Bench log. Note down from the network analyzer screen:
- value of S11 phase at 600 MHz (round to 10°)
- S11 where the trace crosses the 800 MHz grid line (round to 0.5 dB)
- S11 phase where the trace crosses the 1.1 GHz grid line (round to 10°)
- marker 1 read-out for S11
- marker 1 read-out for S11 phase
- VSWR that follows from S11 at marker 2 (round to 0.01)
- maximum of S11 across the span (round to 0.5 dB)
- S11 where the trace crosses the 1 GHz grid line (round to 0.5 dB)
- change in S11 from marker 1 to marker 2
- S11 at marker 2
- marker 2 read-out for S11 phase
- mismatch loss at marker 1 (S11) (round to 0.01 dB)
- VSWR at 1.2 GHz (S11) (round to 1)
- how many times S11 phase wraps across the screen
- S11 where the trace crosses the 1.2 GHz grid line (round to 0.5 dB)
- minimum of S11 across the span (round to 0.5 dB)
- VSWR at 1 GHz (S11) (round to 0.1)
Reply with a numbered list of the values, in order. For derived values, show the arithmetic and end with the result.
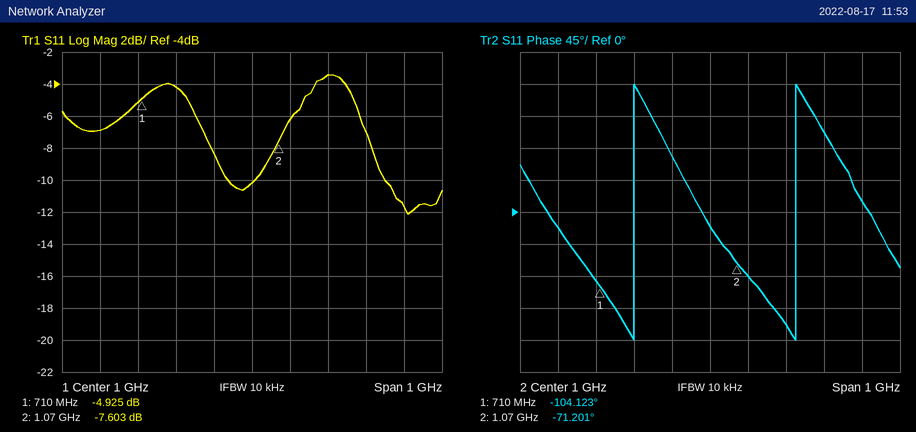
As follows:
1. -20°
2. -4.0 dB
3. -90°
4. -4.925 dB
5. -104.123°
6. (1 + 0.4167)/(1 − 0.4167) ≈ 2.43
7. -3.5 dB
8. -10.0 dB
9. -7.603 − (-4.925) = -2.678 dB
10. -7.603 dB
11. -71.201°
12. −10 log10(1 − 10^(-4.925/10)) ≈ 1.69 dB
13. |Γ| = 10^(-3.5/20) = 0.6683; VSWR = (1 + 0.6683)/(1 − 0.6683) ≈ 5
14. 2
15. -3.5 dB
16. -12.0 dB
17. |Γ| = 10^(-10/20) = 0.3162; VSWR = (1 + 0.3162)/(1 − 0.3162) ≈ 1.9
